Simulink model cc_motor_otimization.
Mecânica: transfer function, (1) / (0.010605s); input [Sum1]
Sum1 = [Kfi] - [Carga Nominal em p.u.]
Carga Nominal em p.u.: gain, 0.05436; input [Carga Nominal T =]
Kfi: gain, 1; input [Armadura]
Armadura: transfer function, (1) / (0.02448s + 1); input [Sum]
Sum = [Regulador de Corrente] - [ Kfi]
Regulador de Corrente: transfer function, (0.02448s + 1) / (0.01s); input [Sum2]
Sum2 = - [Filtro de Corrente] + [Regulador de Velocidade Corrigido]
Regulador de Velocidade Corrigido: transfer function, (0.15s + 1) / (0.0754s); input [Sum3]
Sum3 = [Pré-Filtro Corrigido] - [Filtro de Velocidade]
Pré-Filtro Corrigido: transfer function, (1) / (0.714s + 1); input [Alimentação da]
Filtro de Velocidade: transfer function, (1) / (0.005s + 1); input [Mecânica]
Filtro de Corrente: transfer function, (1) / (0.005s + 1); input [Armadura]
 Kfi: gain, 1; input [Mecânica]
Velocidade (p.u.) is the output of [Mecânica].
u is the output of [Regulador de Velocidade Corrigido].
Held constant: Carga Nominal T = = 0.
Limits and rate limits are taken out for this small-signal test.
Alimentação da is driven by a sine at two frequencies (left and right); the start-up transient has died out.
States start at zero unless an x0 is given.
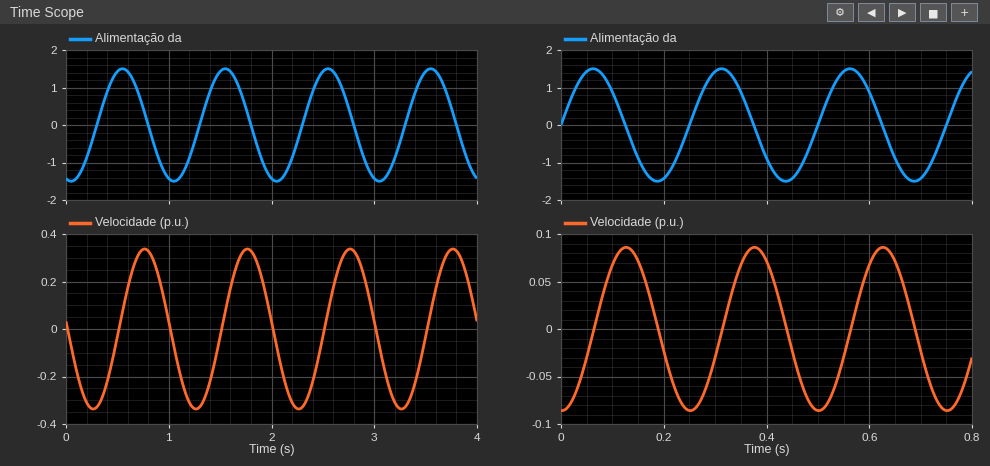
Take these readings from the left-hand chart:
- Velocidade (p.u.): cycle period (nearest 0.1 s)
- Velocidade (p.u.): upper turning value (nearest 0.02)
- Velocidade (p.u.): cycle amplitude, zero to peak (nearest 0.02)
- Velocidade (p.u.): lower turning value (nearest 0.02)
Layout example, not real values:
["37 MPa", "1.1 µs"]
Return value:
["1.0 s", "0.34", "0.34", "-0.34"]
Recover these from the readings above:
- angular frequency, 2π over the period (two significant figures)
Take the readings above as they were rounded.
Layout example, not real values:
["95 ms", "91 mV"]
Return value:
["6.3 rad/s"]
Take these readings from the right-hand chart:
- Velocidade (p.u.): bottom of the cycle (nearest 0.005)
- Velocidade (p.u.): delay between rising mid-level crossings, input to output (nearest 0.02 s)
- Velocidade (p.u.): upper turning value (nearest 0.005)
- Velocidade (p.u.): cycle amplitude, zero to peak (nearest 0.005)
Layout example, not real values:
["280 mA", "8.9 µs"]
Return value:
["-0.085", "0.06 s", "0.085", "0.085"]
